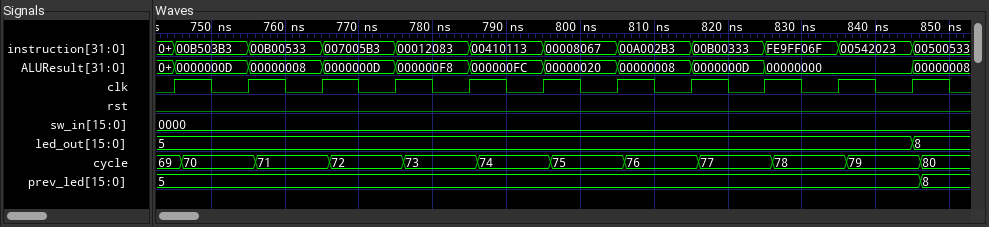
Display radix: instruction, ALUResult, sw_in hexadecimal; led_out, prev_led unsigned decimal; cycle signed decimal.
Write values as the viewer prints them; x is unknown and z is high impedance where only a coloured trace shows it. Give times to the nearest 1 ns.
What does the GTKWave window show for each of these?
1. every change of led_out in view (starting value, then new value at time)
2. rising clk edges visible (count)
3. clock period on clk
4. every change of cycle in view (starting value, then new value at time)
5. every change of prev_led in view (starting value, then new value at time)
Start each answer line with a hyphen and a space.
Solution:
- 5, 8 at 845 ns
- 11
- 10 ns
- 69, 70 at 746 ns, 71 at 756 ns, 72 at 766 ns, 73 at 776 ns, 74 at 786 ns, 75 at 796 ns, 76 at 806 ns, 77 at 816 ns, 78 at 826 ns, 79 at 836 ns, 80 at 846 ns
- 5, 8 at 846 ns
